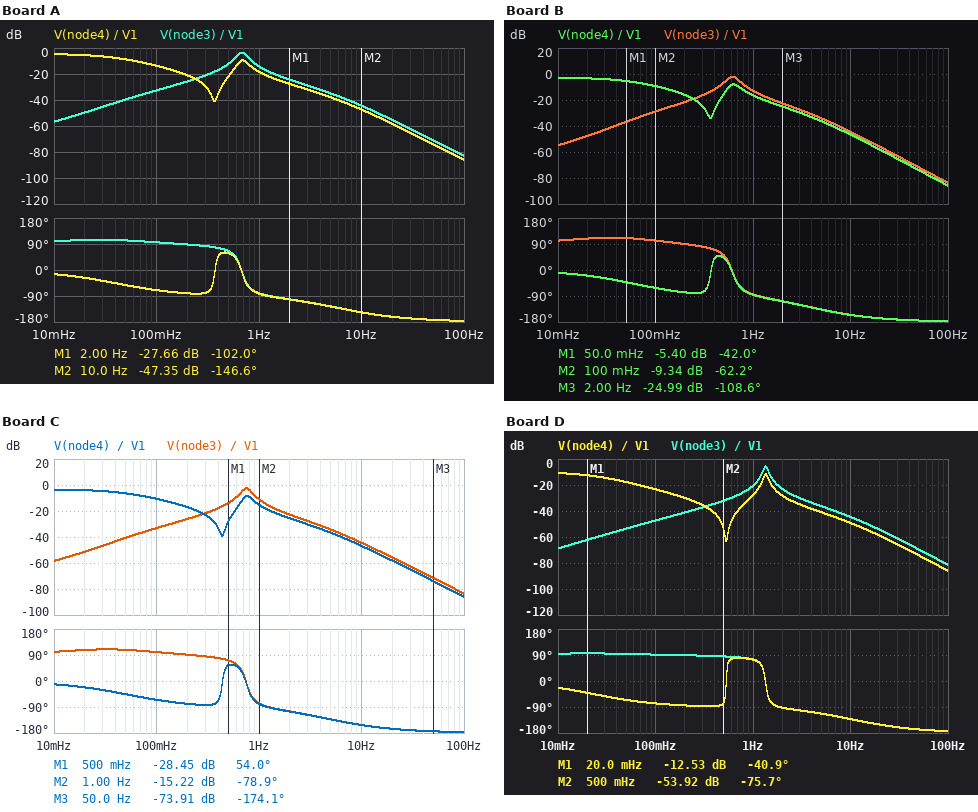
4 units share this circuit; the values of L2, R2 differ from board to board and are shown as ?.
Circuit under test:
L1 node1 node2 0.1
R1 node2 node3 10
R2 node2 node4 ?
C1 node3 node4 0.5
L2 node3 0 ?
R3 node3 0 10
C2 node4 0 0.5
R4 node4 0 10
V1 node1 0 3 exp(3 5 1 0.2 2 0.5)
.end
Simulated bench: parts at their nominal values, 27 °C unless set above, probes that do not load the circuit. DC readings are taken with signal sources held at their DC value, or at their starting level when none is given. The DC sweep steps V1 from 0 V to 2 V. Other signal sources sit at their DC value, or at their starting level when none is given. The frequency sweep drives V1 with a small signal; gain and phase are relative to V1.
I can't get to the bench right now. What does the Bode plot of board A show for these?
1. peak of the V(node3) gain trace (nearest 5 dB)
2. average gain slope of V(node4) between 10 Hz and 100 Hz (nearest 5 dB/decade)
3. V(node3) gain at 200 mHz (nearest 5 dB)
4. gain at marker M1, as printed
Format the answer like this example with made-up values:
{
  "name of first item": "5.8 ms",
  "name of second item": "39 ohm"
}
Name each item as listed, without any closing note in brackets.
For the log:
{
  "peak of the V(node3) gain trace": "-5 dB",
  "average gain slope of V(node4) between 10 Hz and 100 Hz": "-40 dB/decade",
  "V(node3) gain at 200 mHz": "-25 dB",
  "gain at marker M1, as printed": "-27.66 dB"
}
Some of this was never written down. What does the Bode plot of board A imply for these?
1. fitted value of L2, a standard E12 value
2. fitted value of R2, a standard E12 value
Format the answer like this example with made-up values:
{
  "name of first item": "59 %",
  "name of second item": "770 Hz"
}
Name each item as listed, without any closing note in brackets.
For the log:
{
  "fitted value of L2, a standard E12 value": "220 mH",
  "fitted value of R2, a standard E12 value": "6.8 Ω"
}
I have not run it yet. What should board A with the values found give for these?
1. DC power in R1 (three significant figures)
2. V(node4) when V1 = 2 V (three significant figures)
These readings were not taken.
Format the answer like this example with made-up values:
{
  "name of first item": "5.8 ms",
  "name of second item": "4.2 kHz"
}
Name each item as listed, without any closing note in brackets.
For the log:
{
  "DC power in R1": "900 mW",
  "V(node4) when V1 = 2 V": "1.19 V"
}
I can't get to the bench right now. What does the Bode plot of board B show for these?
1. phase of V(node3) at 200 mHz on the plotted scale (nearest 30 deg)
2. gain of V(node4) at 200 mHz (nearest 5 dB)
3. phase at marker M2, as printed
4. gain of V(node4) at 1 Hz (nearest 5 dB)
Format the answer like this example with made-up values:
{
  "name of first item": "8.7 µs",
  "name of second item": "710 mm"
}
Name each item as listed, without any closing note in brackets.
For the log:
{
  "phase of V(node3) at 200 mHz on the plotted scale": "90 deg",
  "gain of V(node4) at 200 mHz": "-15 dB",
  "phase at marker M2, as printed": "-62.2 deg",
  "gain of V(node4) at 1 Hz": "-15 dB"
}
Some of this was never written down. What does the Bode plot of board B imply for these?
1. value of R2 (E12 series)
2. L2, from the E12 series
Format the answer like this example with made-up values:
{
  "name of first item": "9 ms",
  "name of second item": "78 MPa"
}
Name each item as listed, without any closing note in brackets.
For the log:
{
  "value of R2": "3.9 Ω",
  "L2, from the E12 series": "270 mH"
}
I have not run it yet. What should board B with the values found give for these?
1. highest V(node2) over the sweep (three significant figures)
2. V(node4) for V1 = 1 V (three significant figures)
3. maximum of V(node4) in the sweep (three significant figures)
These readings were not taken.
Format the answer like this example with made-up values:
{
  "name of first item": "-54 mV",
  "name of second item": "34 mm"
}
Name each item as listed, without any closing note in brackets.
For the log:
{
  "highest V(node2) over the sweep": "2.00 V",
  "V(node4) for V1 = 1 V": "719 mV",
  "maximum of V(node4) in the sweep": "1.44 V"
}
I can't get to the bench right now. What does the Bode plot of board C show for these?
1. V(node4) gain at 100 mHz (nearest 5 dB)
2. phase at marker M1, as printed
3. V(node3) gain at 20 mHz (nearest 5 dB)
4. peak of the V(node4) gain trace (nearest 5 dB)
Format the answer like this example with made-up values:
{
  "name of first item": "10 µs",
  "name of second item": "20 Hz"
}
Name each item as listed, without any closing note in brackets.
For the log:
{
  "V(node4) gain at 100 mHz": "-10 dB",
  "phase at marker M1, as printed": "54.0 deg",
  "V(node3) gain at 20 mHz": "-50 dB",
  "peak of the V(node4) gain trace": "-5 dB"
}
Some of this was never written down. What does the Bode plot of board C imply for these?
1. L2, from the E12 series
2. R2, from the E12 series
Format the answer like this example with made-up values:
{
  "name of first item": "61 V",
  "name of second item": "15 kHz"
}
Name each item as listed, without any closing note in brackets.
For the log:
{
  "L2, from the E12 series": "180 mH",
  "R2, from the E12 series": "4.7 Ω"
}
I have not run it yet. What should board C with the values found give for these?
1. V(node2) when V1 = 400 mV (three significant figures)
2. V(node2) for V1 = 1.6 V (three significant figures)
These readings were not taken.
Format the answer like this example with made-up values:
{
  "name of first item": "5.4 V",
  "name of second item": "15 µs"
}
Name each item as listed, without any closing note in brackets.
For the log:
{
  "V(node2) when V1 = 400 mV": "400 mV",
  "V(node2) for V1 = 1.6 V": "1.60 V"
}
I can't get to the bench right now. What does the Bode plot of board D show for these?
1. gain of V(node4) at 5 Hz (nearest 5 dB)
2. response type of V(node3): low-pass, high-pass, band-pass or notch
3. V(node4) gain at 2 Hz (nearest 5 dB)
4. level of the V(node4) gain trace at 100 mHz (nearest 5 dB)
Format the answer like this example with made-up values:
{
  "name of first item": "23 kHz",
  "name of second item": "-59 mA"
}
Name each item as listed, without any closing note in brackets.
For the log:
{
  "gain of V(node4) at 5 Hz": "-40 dB",
  "response type of V(node3): low-pass, high-pass, band-pass or notch": "band-pass",
  "V(node4) gain at 2 Hz": "-30 dB",
  "level of the V(node4) gain trace at 100 mHz": "-25 dB"
}
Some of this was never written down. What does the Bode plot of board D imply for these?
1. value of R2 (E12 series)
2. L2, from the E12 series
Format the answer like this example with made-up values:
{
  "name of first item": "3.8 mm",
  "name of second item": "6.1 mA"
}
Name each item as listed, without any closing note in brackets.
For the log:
{
  "value of R2": "22 Ω",
  "L2, from the E12 series": "56 mH"
}
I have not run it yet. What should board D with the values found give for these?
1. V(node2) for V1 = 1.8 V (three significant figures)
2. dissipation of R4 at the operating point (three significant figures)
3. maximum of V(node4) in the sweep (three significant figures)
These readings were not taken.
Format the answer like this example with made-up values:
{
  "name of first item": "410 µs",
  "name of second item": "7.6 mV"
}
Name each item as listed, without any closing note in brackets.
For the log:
{
  "V(node2) for V1 = 1.8 V": "1.80 V",
  "dissipation of R4 at the operating point": "87.9 mW",
  "maximum of V(node4) in the sweep": "625 mV"
}
